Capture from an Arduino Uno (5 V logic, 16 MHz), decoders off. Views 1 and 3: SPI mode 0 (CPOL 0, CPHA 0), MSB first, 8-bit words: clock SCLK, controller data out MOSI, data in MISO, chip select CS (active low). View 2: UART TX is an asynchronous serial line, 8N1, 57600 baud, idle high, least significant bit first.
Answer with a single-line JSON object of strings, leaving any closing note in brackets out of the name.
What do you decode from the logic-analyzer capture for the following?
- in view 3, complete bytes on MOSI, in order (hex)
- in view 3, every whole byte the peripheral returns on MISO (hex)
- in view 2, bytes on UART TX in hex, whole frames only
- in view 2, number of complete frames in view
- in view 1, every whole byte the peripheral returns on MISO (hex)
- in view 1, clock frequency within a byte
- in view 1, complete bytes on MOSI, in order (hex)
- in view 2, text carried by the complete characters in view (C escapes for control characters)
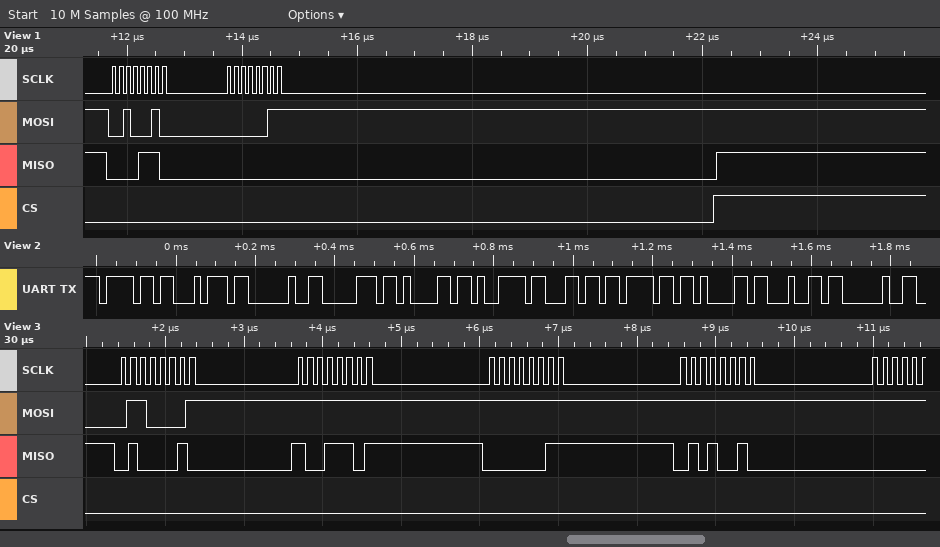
{"in view 3, complete bytes on MOSI, in order": "61 FF FF FF", "in view 3, every whole byte the peripheral returns on MISO": "42 9D 03 52", "in view 2, bytes on UART TX in hex, whole frames only": "0x6F 0x74 0x20 0x70 0x61 0x79 0x6C 0x6F 0x61 0x64 0x20", "in view 2, number of complete frames in view": "11", "in view 1, every whole byte the peripheral returns on MISO": "0E 00", "in view 1, clock frequency within a byte": "8 MHz", "in view 1, complete bytes on MOSI, in order": "22 03", "in view 2, text carried by the complete characters in view": "\"ot payload \""}
